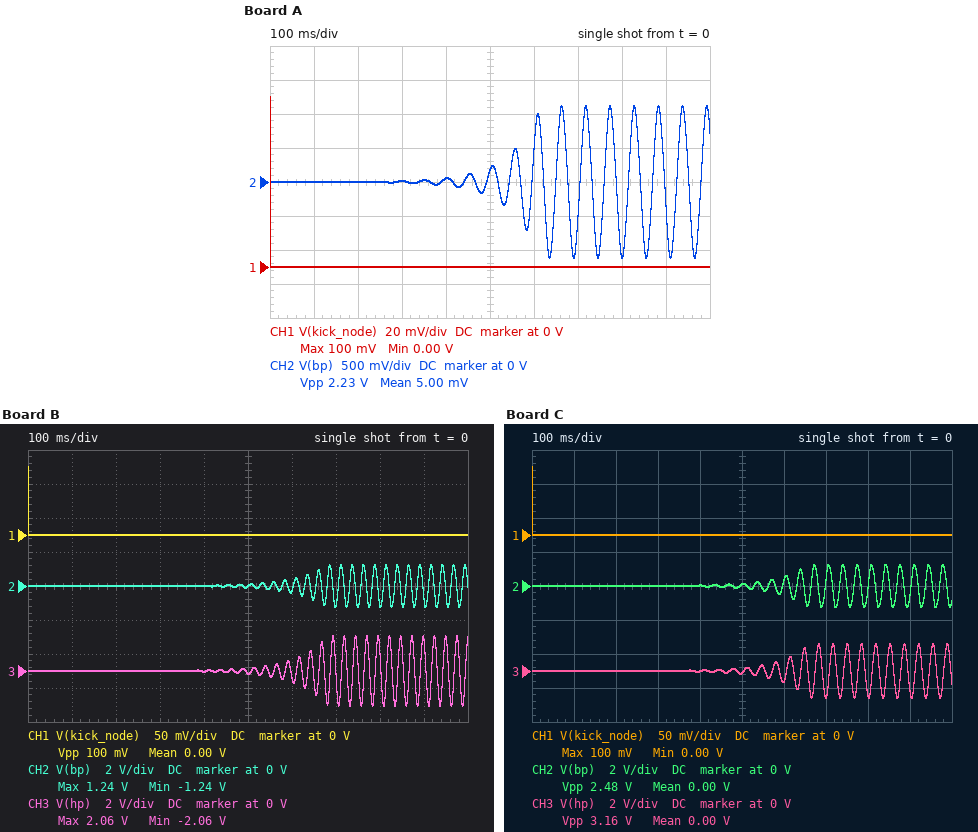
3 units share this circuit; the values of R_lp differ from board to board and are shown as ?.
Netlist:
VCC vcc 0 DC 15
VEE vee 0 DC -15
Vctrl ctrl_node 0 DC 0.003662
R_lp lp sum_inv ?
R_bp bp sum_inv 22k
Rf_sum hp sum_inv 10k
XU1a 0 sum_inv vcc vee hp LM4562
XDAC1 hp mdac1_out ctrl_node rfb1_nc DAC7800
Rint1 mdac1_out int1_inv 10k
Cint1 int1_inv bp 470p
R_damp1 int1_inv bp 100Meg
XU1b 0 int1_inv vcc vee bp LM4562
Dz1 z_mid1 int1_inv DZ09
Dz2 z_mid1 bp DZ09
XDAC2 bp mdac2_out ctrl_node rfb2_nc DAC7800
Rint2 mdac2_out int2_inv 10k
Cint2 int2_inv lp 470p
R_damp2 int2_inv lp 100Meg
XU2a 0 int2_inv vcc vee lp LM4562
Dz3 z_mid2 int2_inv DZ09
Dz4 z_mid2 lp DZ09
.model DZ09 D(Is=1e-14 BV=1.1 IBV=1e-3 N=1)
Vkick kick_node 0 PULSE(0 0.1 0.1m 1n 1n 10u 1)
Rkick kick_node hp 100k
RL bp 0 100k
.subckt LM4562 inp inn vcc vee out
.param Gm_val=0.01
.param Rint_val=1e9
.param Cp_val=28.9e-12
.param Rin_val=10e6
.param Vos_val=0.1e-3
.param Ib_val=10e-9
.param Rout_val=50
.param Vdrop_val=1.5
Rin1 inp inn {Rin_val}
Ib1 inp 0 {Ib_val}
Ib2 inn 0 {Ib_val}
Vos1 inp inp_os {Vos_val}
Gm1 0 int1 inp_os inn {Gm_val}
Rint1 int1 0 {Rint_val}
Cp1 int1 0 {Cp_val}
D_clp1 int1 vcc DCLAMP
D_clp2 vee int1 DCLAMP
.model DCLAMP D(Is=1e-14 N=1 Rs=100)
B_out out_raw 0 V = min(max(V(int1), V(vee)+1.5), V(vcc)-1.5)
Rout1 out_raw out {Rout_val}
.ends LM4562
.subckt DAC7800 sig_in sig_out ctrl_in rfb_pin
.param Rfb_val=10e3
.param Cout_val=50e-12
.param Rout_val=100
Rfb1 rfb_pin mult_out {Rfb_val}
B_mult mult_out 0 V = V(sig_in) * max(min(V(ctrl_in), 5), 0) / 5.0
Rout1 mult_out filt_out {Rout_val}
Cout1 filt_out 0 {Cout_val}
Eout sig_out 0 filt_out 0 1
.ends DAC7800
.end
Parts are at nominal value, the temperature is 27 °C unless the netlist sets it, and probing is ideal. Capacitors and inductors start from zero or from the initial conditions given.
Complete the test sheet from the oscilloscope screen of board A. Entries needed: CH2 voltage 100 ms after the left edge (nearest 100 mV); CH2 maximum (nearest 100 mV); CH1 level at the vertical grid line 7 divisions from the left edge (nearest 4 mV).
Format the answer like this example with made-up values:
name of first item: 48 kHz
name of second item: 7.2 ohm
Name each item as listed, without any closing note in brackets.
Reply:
CH2 voltage 100 ms after the left edge: 0 V
CH2 maximum: 1.1 V
CH1 level at the vertical grid line 7 divisions from the left edge: 0 V
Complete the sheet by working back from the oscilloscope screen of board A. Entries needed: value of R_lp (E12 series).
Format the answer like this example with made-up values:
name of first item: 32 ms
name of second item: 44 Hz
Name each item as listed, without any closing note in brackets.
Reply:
value of R_lp: 15 kΩ
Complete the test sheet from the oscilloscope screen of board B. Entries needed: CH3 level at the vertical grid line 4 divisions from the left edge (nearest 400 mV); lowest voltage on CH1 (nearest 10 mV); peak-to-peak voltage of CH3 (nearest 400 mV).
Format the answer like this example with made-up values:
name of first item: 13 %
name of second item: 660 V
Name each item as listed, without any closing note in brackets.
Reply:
CH3 level at the vertical grid line 4 divisions from the left edge: 0 V
lowest voltage on CH1: 0 V
peak-to-peak voltage of CH3: 4.0 V
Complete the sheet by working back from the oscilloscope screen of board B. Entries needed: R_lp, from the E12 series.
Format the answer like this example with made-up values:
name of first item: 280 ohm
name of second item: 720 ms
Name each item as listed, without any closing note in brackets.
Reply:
R_lp, from the E12 series: 3.9 kΩ
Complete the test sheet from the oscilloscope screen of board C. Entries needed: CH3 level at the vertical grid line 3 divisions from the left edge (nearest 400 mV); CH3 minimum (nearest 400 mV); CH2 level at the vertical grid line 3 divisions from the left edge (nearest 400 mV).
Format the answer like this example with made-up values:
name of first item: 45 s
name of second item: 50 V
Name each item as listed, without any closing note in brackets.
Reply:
CH3 level at the vertical grid line 3 divisions from the left edge: 0 V
CH3 minimum: -1.6 V
CH2 level at the vertical grid line 3 divisions from the left edge: 0 V
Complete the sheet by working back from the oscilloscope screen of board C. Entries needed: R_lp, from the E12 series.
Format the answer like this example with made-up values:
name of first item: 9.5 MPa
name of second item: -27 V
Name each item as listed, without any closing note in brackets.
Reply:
R_lp, from the E12 series: 6.8 kΩ
